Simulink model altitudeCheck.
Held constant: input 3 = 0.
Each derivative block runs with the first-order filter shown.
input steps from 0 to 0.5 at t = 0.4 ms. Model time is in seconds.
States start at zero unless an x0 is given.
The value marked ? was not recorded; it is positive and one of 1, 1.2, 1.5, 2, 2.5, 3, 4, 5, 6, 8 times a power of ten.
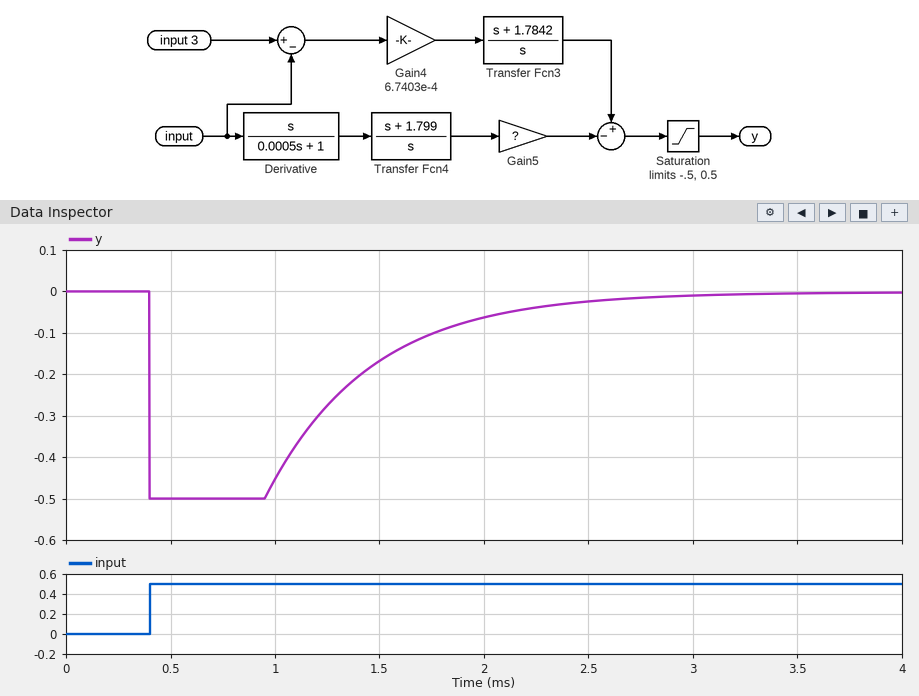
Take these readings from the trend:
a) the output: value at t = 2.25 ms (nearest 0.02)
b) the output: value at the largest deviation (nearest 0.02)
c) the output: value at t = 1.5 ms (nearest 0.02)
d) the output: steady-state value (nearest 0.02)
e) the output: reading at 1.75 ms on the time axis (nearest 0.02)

-0.04
-0.50
-0.16
0.00
-0.10
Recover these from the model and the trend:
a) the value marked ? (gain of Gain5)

0.0015
